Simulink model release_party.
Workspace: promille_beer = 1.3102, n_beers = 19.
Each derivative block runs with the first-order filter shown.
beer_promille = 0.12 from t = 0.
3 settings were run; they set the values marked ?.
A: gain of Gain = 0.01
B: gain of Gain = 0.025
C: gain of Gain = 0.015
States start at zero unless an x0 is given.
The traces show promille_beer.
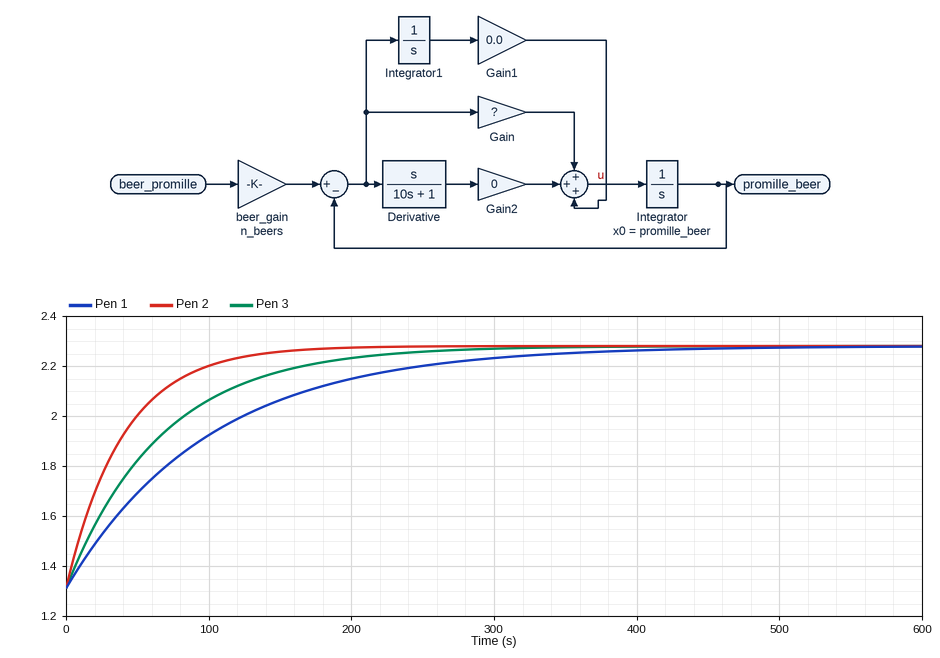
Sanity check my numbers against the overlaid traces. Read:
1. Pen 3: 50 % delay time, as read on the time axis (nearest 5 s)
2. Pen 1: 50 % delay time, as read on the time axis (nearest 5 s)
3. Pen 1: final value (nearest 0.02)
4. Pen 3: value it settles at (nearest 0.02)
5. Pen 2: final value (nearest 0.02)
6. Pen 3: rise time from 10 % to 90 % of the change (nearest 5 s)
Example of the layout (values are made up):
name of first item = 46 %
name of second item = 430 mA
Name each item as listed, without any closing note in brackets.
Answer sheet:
Pen 3: 50 % delay time, as read on the time axis = 45 s
Pen 1: 50 % delay time, as read on the time axis = 70 s
Pen 1: final value = 2.28
Pen 3: value it settles at = 2.28
Pen 2: final value = 2.28
Pen 3: rise time from 10 % to 90 % of the change = 145 s
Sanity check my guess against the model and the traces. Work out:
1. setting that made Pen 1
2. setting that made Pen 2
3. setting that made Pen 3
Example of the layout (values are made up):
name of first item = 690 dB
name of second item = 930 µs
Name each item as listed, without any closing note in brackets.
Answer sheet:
setting that made Pen 1 = A
setting that made Pen 2 = B
setting that made Pen 3 = C
